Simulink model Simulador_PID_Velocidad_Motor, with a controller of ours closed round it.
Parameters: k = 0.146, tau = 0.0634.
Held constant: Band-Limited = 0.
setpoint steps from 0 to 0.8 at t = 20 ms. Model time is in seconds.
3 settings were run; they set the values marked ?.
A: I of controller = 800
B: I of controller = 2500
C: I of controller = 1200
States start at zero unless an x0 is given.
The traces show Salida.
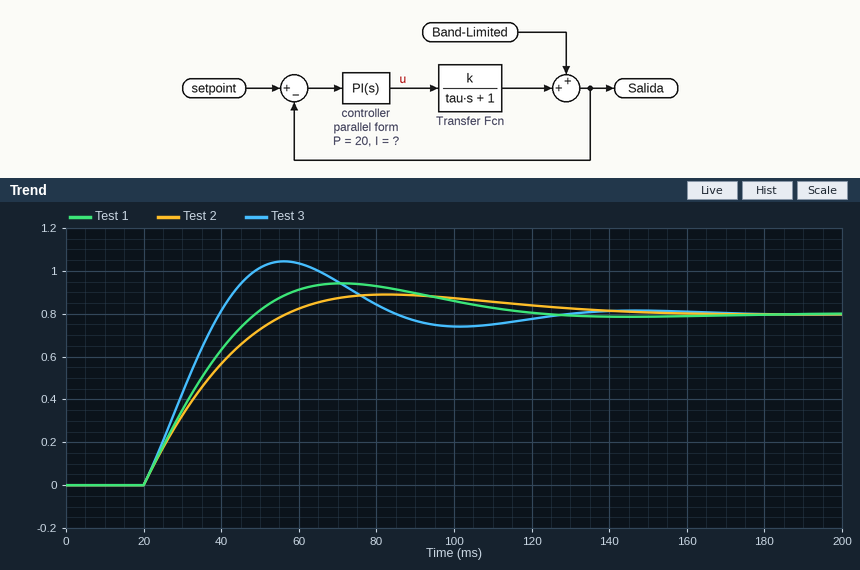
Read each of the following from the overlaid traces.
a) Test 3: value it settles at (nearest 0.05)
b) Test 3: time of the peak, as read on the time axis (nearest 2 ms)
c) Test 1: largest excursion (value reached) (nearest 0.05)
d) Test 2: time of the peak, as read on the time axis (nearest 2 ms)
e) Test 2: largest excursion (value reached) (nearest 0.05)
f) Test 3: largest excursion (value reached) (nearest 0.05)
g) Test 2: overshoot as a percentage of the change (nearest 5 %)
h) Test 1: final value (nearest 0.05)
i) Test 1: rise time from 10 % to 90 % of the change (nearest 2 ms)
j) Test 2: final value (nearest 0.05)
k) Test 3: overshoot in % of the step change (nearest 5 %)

0.80
56 ms
0.95
82 ms
0.90
1.05
10 %
0.80
22 ms
0.80
30 %
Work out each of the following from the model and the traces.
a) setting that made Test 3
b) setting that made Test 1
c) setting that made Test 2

B
C
A
